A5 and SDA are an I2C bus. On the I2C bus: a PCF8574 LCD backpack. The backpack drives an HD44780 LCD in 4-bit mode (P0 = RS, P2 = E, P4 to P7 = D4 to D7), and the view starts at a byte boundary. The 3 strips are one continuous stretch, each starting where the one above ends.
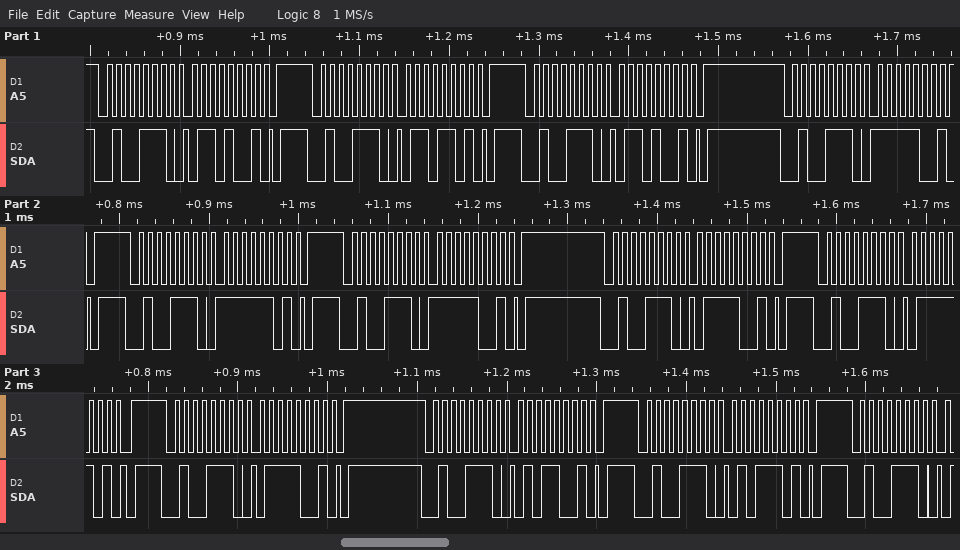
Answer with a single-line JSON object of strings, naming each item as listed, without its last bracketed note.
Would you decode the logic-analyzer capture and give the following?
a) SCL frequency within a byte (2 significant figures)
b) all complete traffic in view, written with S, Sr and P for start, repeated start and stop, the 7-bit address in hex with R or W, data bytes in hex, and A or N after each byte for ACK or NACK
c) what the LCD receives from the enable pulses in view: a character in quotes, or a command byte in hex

{"SCL frequency within a byte": "100 kHz", "all complete traffic in view, written with S, Sr and P for start, repeated start and stop, the 7-bit address in hex with R or W, data bytes in hex, and A or N after each byte for ACK or NACK": "S 27W A 69 A P S 27W A 6D A P S 27W A 69 A P S 27W A F9 A P S 27W A FD A P S 27W A F9 A P S 27W A 79 A P S 27W A 7D A P S 27W A 79 A P S 27W A 59 A P S 27W A 5D A P S 27W A", "what the LCD receives from the enable pulses in view: a character in quotes, or a command byte in hex": "'o'"}
